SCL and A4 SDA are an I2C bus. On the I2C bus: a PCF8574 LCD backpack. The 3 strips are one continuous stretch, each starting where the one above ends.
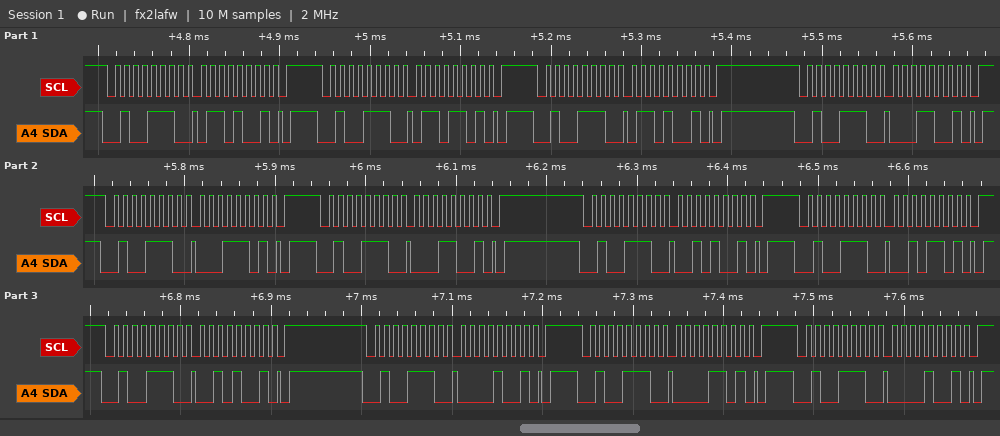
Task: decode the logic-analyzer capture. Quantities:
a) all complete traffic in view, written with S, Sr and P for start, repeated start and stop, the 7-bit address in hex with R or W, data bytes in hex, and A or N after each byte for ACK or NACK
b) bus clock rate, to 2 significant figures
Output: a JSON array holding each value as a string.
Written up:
["S 27W A 69 A P S 27W A 6D A P S 27W A 69 A P S 27W A 19 A P S 27W A 1D A P S 27W A 19 A P S 27W A 29 A P S 27W A 2D A P S 27W A 29 A P S 27W A 09 A P S 27W A 0D A P S 27W A 09 A P", "100 kHz"]
